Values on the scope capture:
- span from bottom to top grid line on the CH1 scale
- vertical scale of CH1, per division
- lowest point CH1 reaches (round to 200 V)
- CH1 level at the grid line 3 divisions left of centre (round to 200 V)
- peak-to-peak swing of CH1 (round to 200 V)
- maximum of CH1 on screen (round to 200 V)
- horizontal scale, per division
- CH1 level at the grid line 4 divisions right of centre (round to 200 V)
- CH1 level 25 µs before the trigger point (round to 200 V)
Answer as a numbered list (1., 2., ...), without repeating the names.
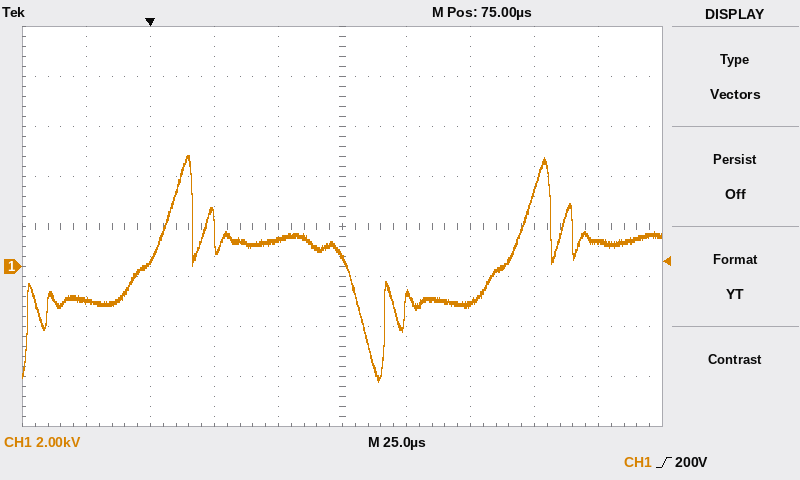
1. 16 kV
2. 2 kV
3. -4.6 kV
4. 200 V
5. 9.0 kV
6. 4.4 kV
7. 25 µs
8. 1.0 kV
9. -1.4 kV
